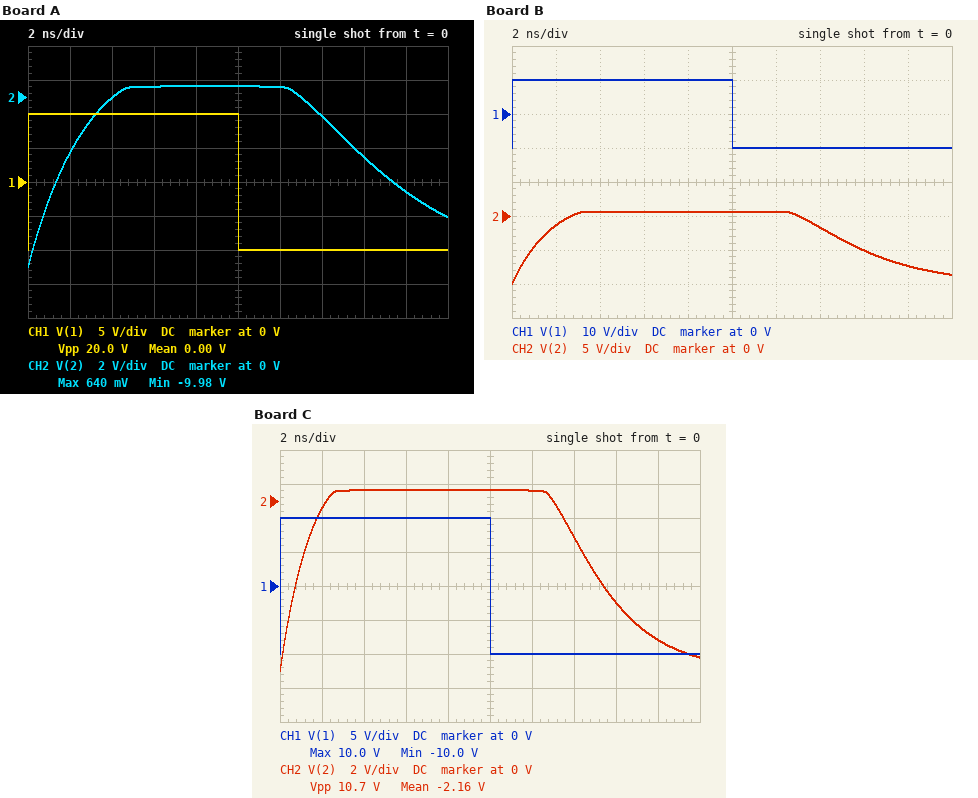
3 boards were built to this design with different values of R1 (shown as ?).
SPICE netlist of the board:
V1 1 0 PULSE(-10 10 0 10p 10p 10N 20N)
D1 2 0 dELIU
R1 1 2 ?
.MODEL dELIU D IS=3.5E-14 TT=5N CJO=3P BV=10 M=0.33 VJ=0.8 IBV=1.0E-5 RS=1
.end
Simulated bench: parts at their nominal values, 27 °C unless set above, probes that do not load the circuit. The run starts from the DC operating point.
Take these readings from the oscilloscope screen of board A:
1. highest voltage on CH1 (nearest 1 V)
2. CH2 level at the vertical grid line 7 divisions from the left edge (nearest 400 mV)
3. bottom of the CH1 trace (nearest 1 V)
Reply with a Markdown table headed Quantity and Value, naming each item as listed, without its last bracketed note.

| Quantity | Value |
|---|---|
| highest voltage on CH1 | 10 V |
| CH2 level at the vertical grid line 7 divisions from the left edge | -1.2 V |
| bottom of the CH1 trace | -10 V |
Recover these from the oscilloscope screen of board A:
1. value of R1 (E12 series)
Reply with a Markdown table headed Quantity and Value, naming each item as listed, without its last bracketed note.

| Quantity | Value |
|---|---|
| value of R1 | 3.3 kΩ |
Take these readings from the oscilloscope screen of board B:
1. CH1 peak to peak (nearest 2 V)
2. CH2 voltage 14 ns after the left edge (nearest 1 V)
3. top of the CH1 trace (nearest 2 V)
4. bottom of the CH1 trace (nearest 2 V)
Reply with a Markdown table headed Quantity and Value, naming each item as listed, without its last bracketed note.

| Quantity | Value |
|---|---|
| CH1 peak to peak | 20 V |
| CH2 voltage 14 ns after the left edge | -2 V |
| top of the CH1 trace | 10 V |
| bottom of the CH1 trace | -10 V |
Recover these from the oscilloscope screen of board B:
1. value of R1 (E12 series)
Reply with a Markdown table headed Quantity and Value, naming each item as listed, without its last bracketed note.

| Quantity | Value |
|---|---|
| value of R1 | 2.2 kΩ |
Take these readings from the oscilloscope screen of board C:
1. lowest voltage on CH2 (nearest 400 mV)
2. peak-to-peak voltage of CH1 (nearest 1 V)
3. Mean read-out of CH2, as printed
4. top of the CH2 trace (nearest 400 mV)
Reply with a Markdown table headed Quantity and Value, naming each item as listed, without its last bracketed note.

| Quantity | Value |
|---|---|
| lowest voltage on CH2 | -10.0 V |
| peak-to-peak voltage of CH1 | 20 V |
| Mean read-out of CH2, as printed | -2.16 V |
| top of the CH2 trace | 800 mV |
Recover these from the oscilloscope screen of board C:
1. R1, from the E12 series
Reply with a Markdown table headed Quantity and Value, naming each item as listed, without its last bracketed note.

| Quantity | Value |
|---|---|
| R1, from the E12 series | 1.8 kΩ |
